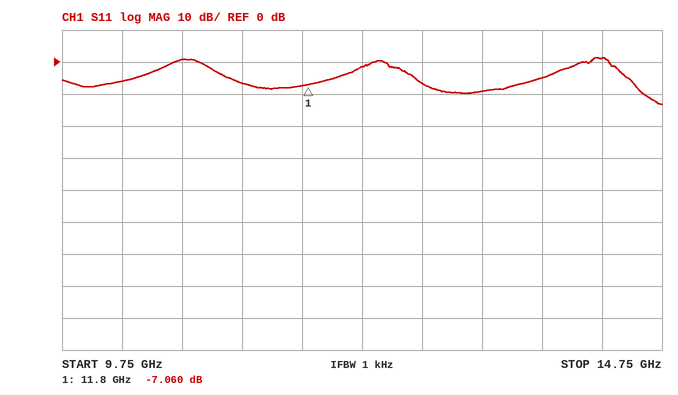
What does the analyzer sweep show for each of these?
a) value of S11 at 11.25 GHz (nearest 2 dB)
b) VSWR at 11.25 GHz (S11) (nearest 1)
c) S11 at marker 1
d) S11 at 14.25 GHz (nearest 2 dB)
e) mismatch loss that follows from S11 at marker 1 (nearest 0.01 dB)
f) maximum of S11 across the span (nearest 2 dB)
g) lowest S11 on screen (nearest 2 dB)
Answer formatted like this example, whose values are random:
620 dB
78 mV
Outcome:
-6 dB
3
-7.060 dB
2 dB
0.95 dB
2 dB
-14 dB
